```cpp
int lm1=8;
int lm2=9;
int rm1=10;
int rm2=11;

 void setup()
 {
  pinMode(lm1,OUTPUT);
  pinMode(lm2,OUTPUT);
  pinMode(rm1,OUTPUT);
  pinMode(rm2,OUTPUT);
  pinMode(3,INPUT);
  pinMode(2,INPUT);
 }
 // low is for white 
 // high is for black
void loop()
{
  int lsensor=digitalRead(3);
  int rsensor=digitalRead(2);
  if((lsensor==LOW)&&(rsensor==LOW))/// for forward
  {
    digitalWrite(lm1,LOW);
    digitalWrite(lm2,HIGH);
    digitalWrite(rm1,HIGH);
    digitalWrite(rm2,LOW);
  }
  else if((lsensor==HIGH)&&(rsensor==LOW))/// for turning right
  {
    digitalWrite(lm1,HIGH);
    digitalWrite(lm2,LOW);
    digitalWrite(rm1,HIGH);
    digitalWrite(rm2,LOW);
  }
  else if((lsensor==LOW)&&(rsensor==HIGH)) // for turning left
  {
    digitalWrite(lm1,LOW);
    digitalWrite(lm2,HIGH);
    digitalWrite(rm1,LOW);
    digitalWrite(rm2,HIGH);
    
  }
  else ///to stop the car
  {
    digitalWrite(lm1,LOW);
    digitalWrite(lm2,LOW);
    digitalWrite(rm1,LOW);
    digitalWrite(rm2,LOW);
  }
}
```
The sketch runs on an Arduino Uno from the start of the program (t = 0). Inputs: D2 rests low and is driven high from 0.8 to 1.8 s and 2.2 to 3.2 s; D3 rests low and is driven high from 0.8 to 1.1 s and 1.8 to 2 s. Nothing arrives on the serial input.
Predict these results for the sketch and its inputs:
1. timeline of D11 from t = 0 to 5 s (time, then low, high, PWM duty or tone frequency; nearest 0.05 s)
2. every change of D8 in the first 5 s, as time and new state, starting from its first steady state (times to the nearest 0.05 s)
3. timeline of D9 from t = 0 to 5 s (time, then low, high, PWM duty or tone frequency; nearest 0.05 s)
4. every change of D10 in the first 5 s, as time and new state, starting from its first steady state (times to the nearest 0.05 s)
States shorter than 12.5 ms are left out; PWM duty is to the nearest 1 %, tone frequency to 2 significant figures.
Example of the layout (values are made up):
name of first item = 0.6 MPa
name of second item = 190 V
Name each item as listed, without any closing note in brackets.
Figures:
timeline of D11 from t = 0 to 5 s = 0 s low; 1.1 s high; 1.8 s low; 2.2 s high; 3.2 s low
every change of D8 in the first 5 s, as time and new state, starting from its first steady state = 0 s low; 1.8 s high; 2 s low
timeline of D9 from t = 0 to 5 s = 0 s high; 0.8 s low; 1.1 s high; 1.8 s low; 2 s high
every change of D10 in the first 5 s, as time and new state, starting from its first steady state = 0 s high; 0.8 s low; 1.8 s high; 2.2 s low; 3.2 s high
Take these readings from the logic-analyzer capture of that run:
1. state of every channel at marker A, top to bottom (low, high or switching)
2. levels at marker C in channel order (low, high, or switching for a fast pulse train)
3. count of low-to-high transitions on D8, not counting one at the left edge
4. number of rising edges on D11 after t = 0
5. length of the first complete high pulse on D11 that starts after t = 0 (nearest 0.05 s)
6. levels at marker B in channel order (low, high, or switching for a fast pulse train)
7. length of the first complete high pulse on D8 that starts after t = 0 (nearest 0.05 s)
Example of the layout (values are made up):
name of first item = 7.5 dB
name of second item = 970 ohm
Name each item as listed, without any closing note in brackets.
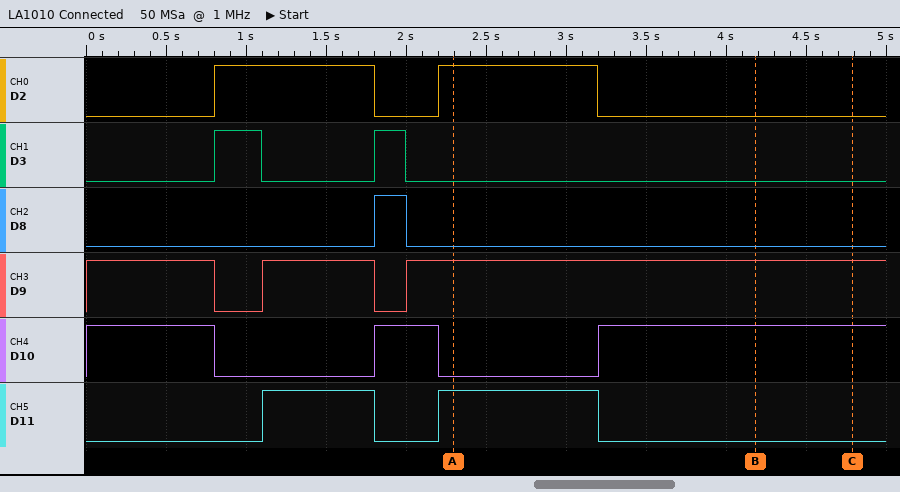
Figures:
state of every channel at marker A, top to bottom = D2 high, D3 low, D8 low, D9 high, D10 low, D11 high
levels at marker C in channel order = D2 low, D3 low, D8 low, D9 high, D10 high, D11 low
count of low-to-high transitions on D8, not counting one at the left edge = 1
number of rising edges on D11 after t = 0 = 2
length of the first complete high pulse on D11 that starts after t = 0 = 0.70 s
levels at marker B in channel order = D2 low, D3 low, D8 low, D9 high, D10 high, D11 low
length of the first complete high pulse on D8 that starts after t = 0 = 0.20 s
